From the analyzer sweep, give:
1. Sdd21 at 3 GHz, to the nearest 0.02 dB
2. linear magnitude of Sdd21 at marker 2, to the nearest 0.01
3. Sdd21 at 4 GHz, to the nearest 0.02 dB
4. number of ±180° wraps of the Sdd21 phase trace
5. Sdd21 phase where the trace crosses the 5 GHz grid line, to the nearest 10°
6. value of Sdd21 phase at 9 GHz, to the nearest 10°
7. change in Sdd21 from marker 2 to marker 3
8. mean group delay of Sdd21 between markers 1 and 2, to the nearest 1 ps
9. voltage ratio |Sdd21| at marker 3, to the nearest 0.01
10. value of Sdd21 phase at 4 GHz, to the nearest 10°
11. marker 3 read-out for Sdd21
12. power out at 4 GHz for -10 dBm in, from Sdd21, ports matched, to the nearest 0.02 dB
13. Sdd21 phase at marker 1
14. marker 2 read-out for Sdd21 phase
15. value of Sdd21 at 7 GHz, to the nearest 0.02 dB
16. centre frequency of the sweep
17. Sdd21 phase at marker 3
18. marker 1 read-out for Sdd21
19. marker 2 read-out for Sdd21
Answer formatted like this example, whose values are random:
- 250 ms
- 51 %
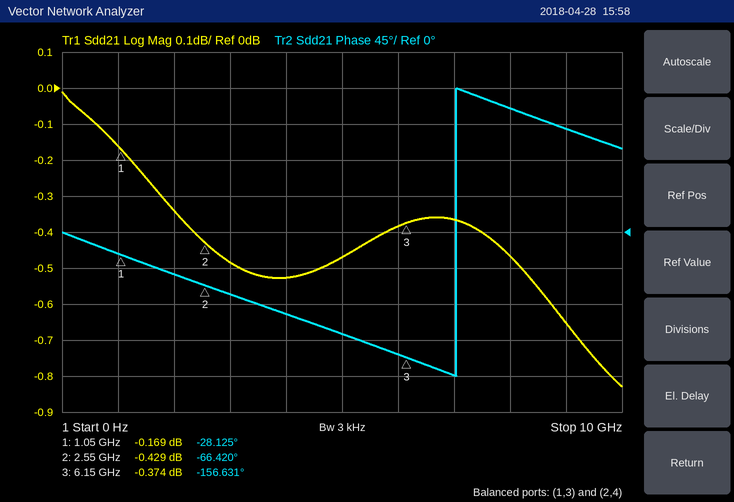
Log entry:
- -0.48 dB
- 0.95
- -0.52 dB
- 1
- -130°
- 130°
- 0.055 dB
- 71 ps
- 0.96
- -100°
- -0.374 dB
- -10.52 dBm
- -28.125°
- -66.420°
- -0.36 dB
- 5 GHz
- -156.631°
- -0.169 dB
- -0.429 dB
